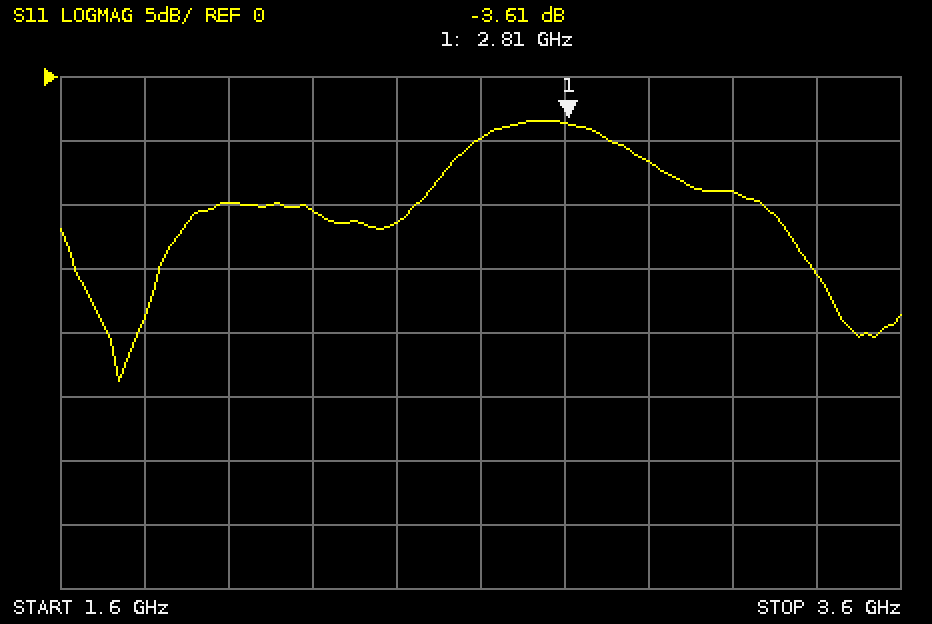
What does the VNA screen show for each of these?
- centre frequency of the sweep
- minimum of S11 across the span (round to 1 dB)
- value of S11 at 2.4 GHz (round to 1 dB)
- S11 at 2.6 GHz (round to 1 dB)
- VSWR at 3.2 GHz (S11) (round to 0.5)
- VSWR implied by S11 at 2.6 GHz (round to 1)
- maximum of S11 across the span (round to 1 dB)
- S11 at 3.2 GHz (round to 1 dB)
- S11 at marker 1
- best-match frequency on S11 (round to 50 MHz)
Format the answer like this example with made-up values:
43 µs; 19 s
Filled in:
2.6 GHz; -24 dB; -11 dB; -5 dB; 2.0; 4; -3 dB; -9 dB; -3.61 dB; 1.75 GHz
